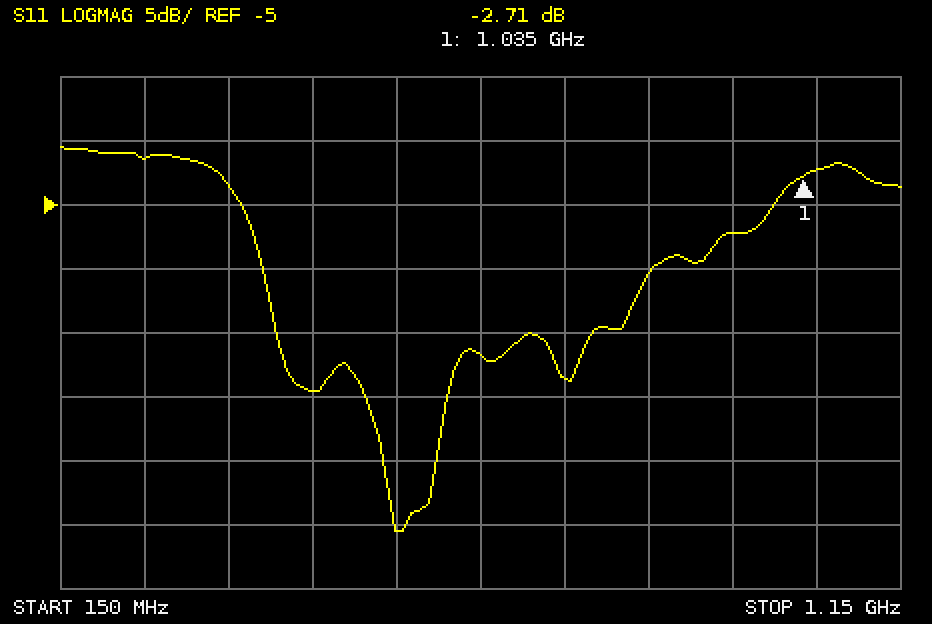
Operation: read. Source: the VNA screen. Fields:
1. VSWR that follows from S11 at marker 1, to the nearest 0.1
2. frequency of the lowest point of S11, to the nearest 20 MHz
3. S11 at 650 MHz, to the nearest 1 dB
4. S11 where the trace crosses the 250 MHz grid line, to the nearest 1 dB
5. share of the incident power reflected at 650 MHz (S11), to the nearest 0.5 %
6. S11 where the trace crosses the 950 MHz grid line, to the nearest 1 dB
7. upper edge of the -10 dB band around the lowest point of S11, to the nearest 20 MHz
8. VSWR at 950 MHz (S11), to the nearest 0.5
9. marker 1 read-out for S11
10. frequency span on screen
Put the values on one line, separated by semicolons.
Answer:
6.5; 540 MHz; -17 dB; -1 dB; 2.0 %; -7 dB; 860 MHz; 2.5; -2.71 dB; 1 GHz
